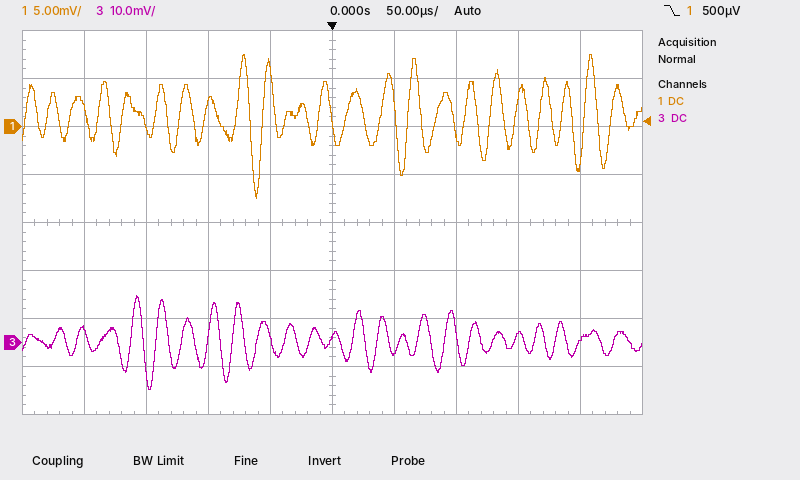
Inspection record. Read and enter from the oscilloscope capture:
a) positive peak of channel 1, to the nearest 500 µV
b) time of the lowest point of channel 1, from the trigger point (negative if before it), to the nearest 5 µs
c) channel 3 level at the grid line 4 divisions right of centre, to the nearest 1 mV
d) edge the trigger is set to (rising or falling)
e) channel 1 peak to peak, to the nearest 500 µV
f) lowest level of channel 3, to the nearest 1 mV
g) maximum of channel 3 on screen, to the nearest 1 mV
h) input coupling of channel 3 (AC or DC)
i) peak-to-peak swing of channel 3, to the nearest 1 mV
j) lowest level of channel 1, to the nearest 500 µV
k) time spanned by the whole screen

7.5 mV
-60 µs
0 mV
falling
15.0 mV
-10 mV
10 mV
DC
20 mV
-7.5 mV
500 µs
